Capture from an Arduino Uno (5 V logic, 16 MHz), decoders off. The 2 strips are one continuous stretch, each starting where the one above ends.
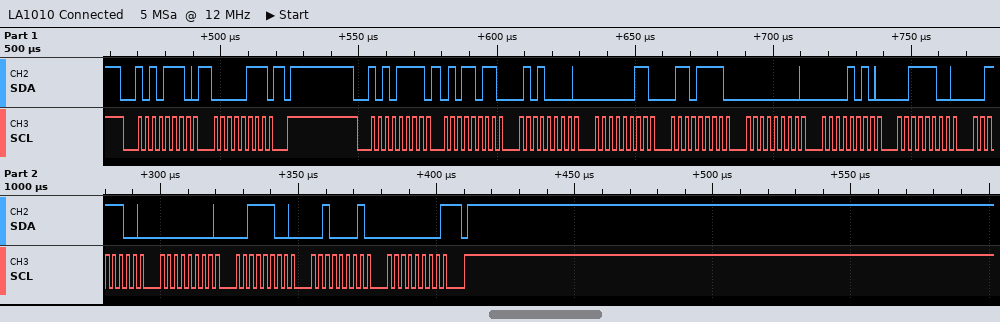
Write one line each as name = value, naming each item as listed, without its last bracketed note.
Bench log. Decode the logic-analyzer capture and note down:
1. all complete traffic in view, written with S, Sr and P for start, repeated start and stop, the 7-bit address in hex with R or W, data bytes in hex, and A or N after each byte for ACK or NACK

all complete traffic in view, written with S, Sr and P for start, repeated start and stop, the 7-bit address in hex with R or W, data bytes in hex, and A or N after each byte for ACK or NACK = S 57W A 07 A P S 57R A 5B A 50 A 03 A 6F A 00 A 0A A 3C A 3C A 00 A 3C A 21 A 00 N P
